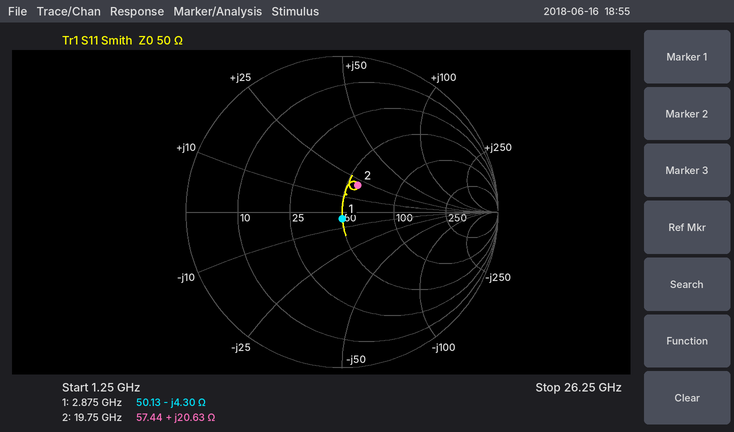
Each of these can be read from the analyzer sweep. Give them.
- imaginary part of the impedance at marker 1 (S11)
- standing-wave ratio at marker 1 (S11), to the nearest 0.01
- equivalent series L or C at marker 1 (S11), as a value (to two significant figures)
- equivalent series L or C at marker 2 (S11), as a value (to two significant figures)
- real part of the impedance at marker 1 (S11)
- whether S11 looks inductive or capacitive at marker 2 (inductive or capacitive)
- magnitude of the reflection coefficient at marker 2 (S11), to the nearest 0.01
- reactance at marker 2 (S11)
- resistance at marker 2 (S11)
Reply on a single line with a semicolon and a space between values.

-4.30 Ω; 1.09; 13 pF; 170 pH; 50.13 Ω; inductive; 0.20; +20.63 Ω; 57.44 Ω
